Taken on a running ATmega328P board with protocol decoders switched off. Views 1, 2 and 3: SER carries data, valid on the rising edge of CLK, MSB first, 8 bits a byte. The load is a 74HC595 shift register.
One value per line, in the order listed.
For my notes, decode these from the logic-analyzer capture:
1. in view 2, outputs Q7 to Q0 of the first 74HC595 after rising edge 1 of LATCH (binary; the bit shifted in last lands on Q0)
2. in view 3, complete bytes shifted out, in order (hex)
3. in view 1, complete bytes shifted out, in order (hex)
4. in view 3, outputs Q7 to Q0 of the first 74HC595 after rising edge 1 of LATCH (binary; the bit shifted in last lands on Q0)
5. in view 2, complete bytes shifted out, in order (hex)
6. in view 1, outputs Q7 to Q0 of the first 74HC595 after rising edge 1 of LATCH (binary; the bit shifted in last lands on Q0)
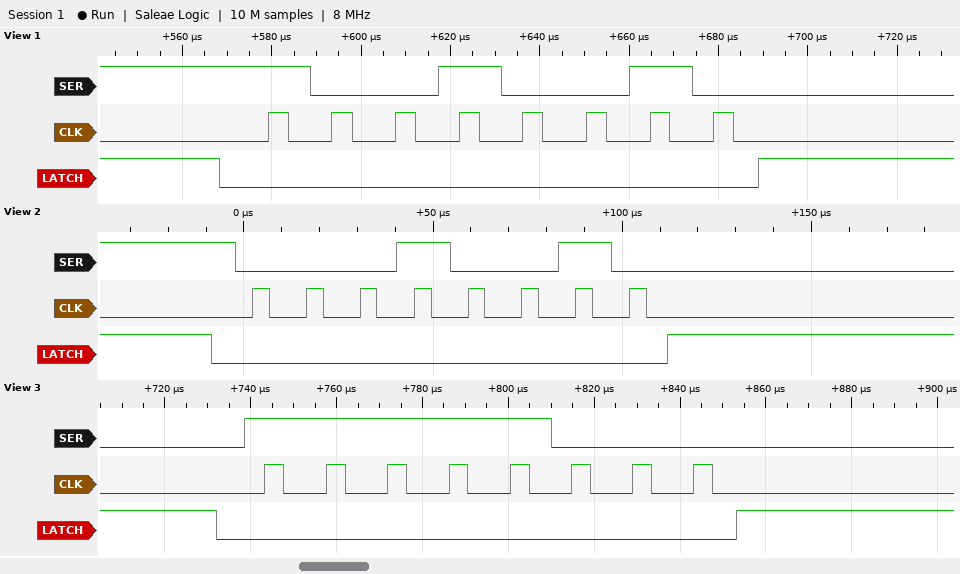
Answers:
00010010
F8
92
11111000
12
10010010
